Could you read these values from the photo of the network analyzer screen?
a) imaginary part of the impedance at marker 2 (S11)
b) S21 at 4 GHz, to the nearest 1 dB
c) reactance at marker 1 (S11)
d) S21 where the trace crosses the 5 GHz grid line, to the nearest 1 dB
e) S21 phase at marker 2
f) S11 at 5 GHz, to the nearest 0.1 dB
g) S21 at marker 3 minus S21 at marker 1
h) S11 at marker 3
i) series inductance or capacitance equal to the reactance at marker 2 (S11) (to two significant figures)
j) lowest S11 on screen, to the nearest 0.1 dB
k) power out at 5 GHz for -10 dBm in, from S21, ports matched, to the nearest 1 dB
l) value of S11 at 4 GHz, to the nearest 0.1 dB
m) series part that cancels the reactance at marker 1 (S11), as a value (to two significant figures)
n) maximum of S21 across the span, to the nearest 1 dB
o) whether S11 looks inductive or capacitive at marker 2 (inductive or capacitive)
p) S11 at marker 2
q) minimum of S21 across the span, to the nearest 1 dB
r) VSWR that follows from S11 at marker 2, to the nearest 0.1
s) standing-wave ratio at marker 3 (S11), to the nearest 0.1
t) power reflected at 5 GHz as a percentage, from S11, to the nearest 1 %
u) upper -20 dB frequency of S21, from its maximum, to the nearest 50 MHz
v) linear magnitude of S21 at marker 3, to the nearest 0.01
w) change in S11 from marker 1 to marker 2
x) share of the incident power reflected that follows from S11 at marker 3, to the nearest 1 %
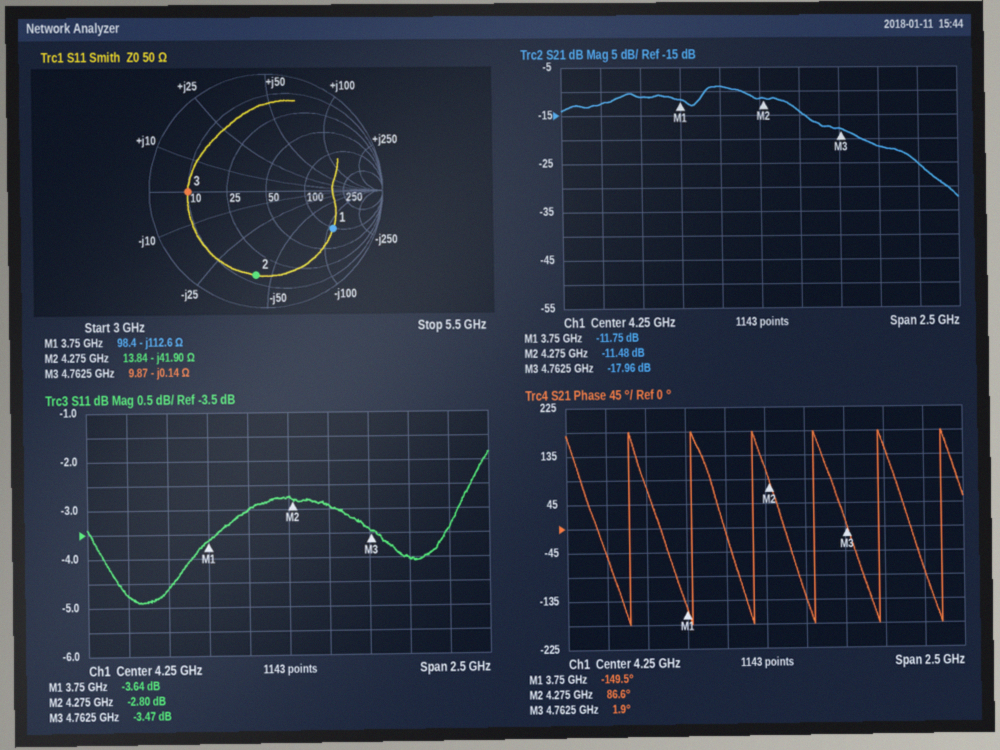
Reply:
-41.90 Ω
-9 dB
-112.6 Ω
-22 dB
86.6°
-4.0 dB
-6.21 dB
-3.47 dB
890 fF
-4.9 dB
-32 dBm
-3.0 dB
4.8 nH
-9 dB
capacitive
-2.80 dB
-32 dB
6.3
5.1
40 %
5.40 GHz
0.13
0.84 dB
45 %
